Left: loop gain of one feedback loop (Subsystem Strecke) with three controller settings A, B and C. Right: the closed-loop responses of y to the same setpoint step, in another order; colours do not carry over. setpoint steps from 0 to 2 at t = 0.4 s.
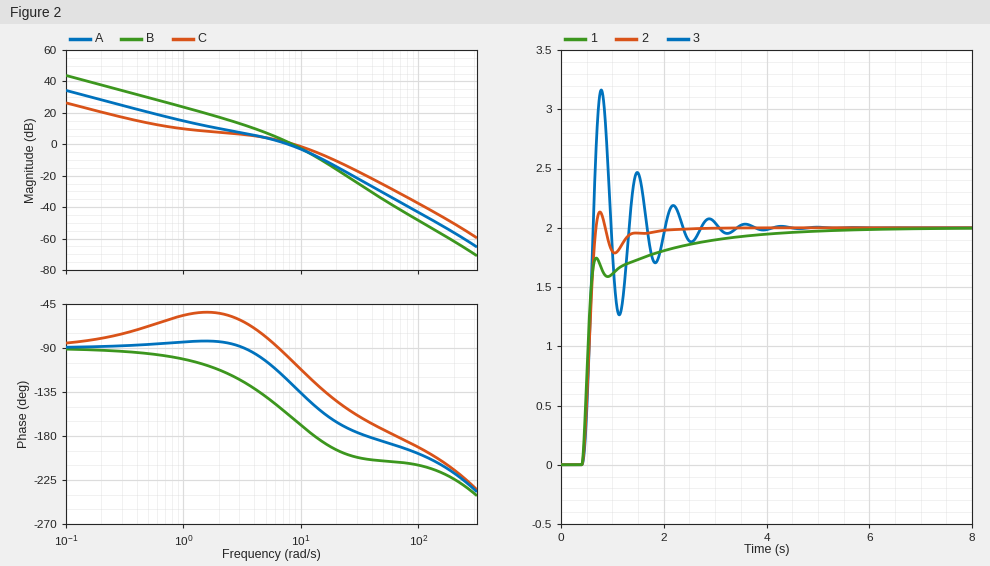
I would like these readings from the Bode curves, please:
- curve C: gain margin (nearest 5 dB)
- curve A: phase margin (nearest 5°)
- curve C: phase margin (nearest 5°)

30 dB
55°
75°
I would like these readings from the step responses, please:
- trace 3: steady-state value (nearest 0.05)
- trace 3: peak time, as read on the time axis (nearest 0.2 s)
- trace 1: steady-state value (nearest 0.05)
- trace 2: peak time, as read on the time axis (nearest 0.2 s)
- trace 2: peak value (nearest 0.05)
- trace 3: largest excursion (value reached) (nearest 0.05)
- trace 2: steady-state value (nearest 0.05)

2.00
0.8 s
2.00
0.8 s
2.15
3.15
2.00
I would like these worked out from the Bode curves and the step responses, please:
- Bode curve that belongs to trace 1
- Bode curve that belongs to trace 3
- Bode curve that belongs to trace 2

C
B
A
